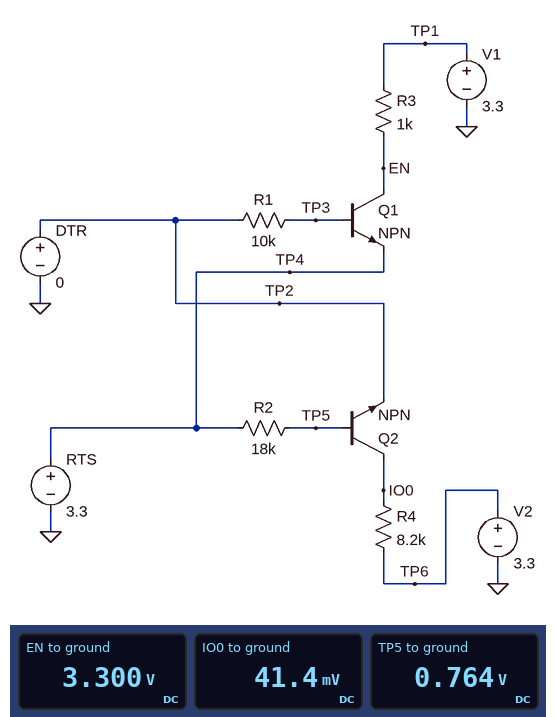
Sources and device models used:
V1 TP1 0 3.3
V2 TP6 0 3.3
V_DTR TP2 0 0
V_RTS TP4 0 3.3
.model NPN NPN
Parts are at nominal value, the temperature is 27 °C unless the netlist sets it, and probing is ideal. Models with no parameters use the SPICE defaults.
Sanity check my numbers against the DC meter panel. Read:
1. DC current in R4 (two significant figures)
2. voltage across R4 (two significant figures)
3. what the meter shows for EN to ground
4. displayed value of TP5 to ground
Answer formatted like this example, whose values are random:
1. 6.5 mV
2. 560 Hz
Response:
1. 400 µA
2. 3.3 V
3. 3.300 V
4. 0.764 V
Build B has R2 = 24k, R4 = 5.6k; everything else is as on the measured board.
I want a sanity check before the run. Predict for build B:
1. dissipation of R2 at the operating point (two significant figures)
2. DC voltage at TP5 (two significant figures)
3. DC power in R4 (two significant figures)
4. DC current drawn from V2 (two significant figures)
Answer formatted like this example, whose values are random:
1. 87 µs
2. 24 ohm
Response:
1. 270 µW
2. 770 mV
3. 1.9 mW
4. 580 µA
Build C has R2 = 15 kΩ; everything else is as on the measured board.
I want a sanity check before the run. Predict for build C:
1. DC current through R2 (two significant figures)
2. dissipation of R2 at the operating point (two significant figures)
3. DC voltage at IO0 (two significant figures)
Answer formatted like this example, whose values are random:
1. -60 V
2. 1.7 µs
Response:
1. 170 µA
2. 430 µW
3. 39 mV
